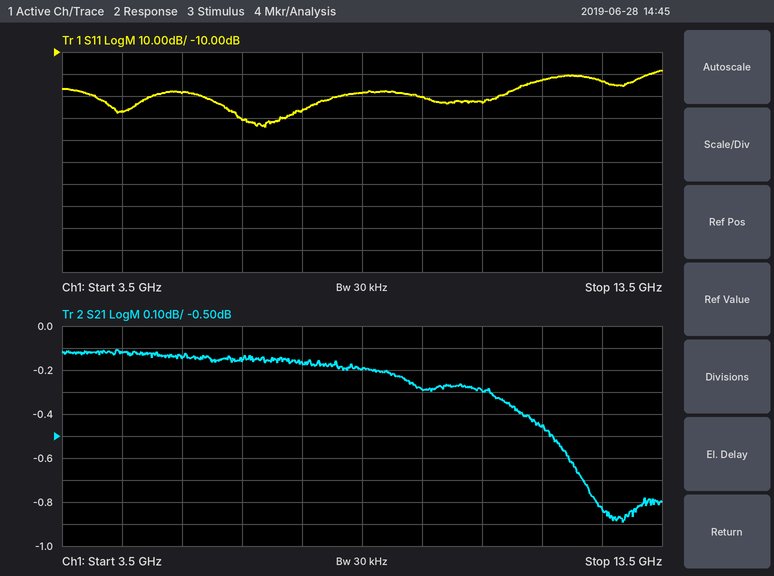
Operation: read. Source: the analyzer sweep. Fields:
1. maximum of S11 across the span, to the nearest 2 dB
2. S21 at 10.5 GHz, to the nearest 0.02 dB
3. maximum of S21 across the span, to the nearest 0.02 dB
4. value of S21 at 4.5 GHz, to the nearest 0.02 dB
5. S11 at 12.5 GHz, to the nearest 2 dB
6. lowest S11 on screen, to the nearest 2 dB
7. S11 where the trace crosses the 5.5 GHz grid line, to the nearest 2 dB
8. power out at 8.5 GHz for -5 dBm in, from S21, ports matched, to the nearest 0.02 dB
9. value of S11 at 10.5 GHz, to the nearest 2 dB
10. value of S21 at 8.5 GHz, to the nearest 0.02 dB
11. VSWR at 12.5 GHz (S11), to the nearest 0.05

-18 dB
-0.30 dB
-0.10 dB
-0.12 dB
-24 dB
-44 dB
-28 dB
-5.20 dBm
-32 dB
-0.20 dB
1.15
